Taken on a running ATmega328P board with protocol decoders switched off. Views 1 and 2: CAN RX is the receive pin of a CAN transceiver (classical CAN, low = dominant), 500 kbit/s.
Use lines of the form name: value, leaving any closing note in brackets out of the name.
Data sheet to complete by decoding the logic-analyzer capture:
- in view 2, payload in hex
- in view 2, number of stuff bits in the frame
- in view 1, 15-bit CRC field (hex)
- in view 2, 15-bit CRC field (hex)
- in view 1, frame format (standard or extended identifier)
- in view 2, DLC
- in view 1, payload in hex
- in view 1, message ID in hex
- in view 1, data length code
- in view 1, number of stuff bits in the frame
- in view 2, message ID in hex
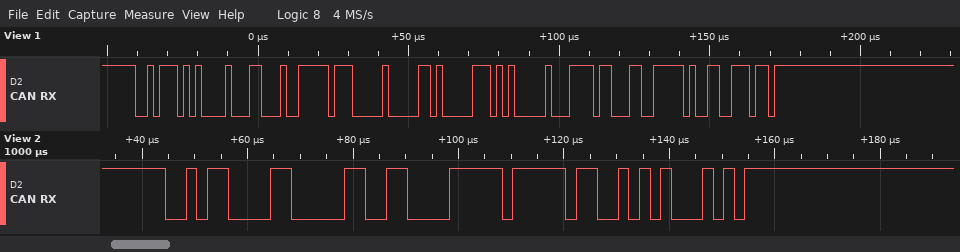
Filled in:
in view 2, payload in hex: 61 FF
in view 2, number of stuff bits in the frame: 3
in view 1, 15-bit CRC field: 0x799D
in view 2, 15-bit CRC field: 0x72A2
in view 1, frame format: standard
in view 2, DLC: 2
in view 1, payload in hex: C4 FF 00 28 35 00 F6 33
in view 1, message ID in hex: 0x2EA
in view 1, data length code: 8
in view 1, number of stuff bits in the frame: 6
in view 2, message ID in hex: 0x2C3
